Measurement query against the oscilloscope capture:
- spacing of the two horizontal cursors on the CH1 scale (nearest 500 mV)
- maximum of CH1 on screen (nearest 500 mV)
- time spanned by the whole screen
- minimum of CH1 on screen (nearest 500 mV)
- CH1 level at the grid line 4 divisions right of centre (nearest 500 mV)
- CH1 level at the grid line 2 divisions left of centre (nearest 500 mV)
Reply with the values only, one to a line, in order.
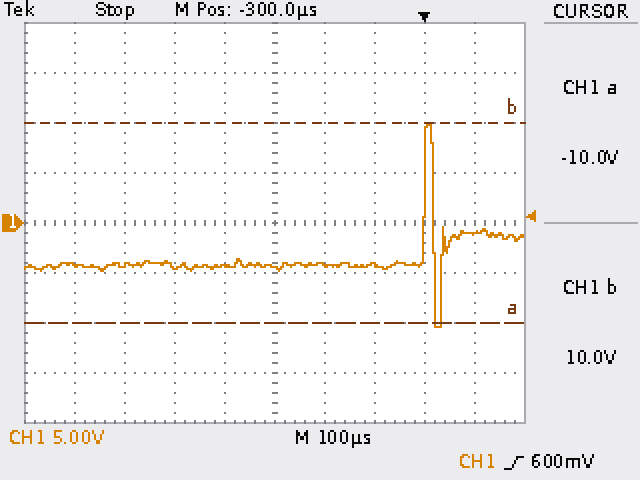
20.0 V
10.0 V
1 ms
-10.5 V
-1.0 V
-4.5 V
